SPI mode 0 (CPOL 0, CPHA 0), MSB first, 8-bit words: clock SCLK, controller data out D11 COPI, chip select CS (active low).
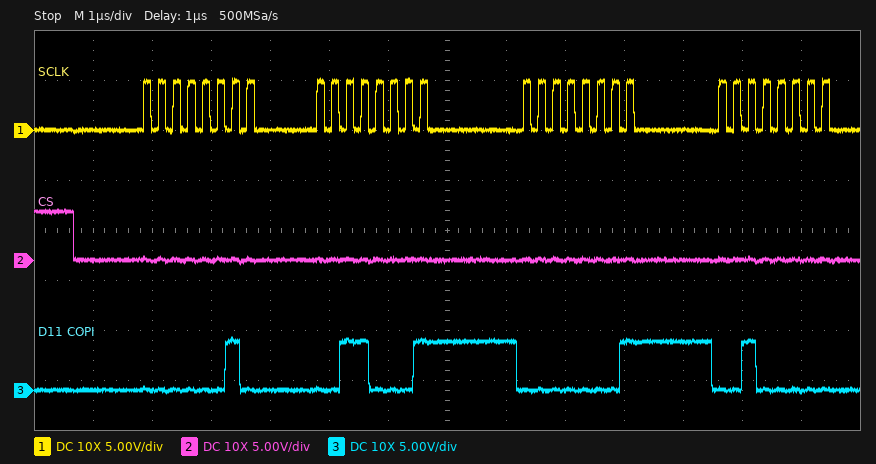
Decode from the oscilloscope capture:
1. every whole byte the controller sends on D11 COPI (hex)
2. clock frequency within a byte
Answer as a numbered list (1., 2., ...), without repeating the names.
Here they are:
1. 02 31 01 20
2. 4 MHz
